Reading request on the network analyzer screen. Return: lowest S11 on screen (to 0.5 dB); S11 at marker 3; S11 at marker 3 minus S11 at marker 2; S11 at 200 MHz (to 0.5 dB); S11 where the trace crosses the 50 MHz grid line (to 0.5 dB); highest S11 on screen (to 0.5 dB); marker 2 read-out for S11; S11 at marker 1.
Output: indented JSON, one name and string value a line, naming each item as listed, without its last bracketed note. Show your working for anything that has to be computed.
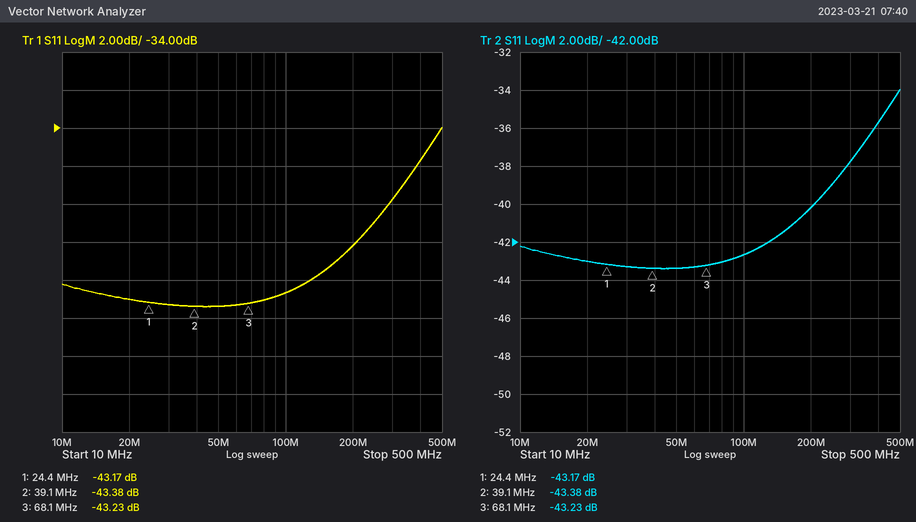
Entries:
{
  "lowest S11 on screen": "-43.5 dB",
  "S11 at marker 3": "-43.23 dB",
  "S11 at marker 3 minus S11 at marker 2": "-43.23 − (-43.38) = 0.15 dB",
  "S11 at 200 MHz": "-40.0 dB",
  "S11 where the trace crosses the 50 MHz grid line": "-43.5 dB",
  "highest S11 on screen": "-34.0 dB",
  "marker 2 read-out for S11": "-43.38 dB",
  "S11 at marker 1": "-43.17 dB"
}
